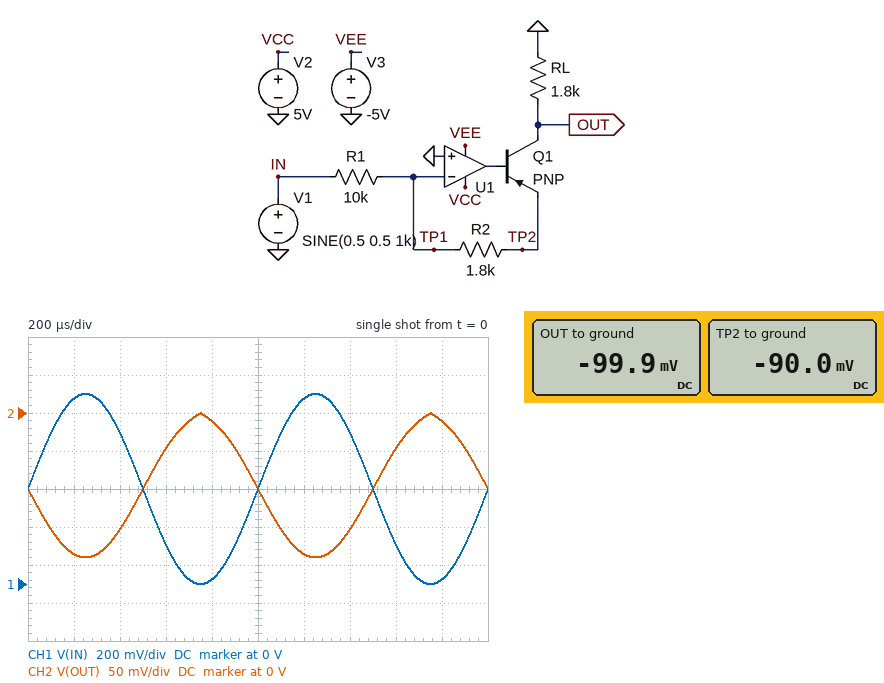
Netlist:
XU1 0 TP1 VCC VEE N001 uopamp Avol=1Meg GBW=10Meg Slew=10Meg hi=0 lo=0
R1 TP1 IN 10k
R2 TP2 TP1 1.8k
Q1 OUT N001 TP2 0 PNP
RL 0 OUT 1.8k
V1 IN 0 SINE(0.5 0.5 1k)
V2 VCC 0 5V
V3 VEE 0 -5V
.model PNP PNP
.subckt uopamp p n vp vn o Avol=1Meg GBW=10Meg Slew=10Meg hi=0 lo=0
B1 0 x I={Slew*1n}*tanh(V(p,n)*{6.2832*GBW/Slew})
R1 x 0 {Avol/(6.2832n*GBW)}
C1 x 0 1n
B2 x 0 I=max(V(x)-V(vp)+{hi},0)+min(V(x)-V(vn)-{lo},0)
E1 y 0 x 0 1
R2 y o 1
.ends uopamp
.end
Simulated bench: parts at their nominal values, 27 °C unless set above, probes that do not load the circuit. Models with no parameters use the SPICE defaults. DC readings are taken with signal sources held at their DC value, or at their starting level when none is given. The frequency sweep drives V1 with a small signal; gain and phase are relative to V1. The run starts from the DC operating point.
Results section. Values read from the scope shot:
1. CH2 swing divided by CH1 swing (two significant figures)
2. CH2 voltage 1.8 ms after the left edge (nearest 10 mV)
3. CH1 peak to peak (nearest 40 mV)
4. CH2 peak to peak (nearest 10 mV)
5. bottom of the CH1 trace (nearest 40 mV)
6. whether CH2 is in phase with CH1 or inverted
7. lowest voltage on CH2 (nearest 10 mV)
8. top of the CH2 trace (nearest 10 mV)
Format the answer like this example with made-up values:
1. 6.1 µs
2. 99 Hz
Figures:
1. 0.19
2. -10 mV
3. 1.00 V
4. 190 mV
5. 0 V
6. inverted
7. -190 mV
8. 0 V
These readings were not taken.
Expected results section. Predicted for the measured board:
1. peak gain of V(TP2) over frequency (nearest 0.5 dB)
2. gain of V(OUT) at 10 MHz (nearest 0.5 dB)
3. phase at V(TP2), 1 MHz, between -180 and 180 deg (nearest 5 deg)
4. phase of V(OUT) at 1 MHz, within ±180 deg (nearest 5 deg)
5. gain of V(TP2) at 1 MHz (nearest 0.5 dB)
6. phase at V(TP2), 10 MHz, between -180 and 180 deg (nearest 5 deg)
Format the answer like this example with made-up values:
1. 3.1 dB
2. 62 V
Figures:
1. -15.0 dB
2. -19.0 dB
3. 170 deg
4. 170 deg
5. -15.0 dB
6. 115 deg
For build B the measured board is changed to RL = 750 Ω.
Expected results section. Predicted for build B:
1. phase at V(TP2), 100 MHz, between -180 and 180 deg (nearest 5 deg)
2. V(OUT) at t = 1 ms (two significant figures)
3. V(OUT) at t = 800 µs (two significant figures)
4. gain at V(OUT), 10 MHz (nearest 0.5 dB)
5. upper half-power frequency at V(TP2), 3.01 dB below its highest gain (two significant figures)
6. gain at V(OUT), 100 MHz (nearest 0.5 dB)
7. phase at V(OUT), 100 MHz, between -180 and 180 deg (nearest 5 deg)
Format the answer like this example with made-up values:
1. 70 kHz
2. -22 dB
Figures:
1. 40 deg
2. -96 mV
3. -8.4 mV
4. -19.5 dB
5. 7.3 MHz
6. -35.5 dB
7. 55 deg
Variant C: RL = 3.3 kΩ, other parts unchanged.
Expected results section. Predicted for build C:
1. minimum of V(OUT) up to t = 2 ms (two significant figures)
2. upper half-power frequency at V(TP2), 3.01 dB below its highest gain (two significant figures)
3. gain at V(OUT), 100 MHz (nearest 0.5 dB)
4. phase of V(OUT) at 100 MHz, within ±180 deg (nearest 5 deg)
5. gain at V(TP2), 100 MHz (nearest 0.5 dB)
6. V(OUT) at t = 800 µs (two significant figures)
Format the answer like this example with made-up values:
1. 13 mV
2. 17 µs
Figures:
1. -190 mV
2. 8.0 MHz
3. -31.0 dB
4. 35 deg
5. -29.5 dB
6. -13 mV
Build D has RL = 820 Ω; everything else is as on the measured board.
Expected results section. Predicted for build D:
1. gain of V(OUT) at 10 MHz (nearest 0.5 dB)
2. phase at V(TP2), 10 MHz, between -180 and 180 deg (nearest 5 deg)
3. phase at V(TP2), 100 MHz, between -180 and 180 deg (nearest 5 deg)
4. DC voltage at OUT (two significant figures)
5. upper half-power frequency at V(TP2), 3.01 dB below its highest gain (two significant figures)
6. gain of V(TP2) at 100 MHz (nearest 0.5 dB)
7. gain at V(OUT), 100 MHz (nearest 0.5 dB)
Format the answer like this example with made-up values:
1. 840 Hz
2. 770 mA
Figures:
1. -19.5 dB
2. 120 deg
3. 40 deg
4. -97 mV
5. 7.4 MHz
6. -33.0 dB
7. -35.5 dB
